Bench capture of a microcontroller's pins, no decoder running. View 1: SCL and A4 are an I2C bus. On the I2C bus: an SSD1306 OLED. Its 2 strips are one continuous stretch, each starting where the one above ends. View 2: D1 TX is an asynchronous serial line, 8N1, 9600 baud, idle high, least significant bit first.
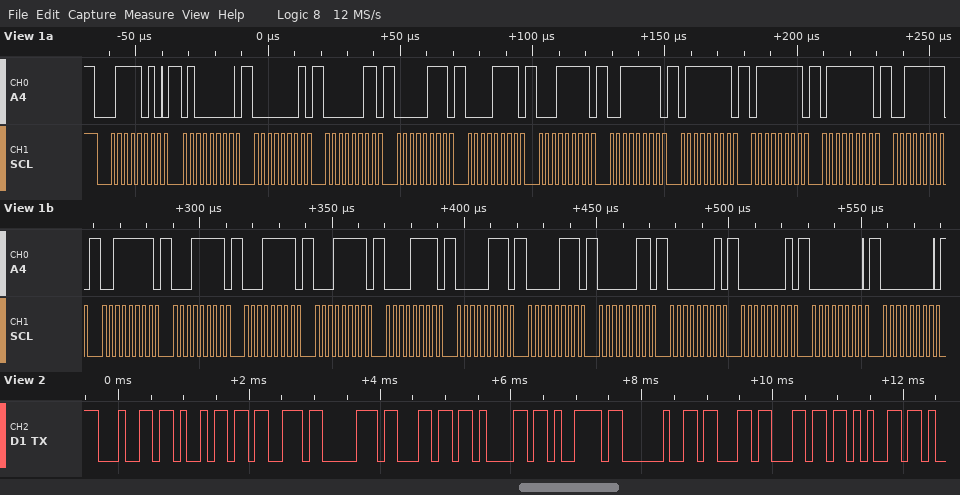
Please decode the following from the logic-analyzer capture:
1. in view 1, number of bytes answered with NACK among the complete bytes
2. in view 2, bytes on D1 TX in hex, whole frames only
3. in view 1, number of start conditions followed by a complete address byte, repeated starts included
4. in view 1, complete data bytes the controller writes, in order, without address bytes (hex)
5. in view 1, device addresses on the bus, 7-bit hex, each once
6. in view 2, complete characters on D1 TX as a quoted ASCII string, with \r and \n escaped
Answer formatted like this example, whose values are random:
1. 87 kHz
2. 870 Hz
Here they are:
1. 0
2. 0x64 0x69 0x73 0x70 0x6C 0x61 0x79 0x20 0x63 0x6C 0x65
3. 1
4. 40 01 03 07 0F 1F 3F 7F 7F 7F 3F 3F 1F 1F 1F 0F 07 07 03 01 01 00 00
5. 0x3D
6. "display cle"
